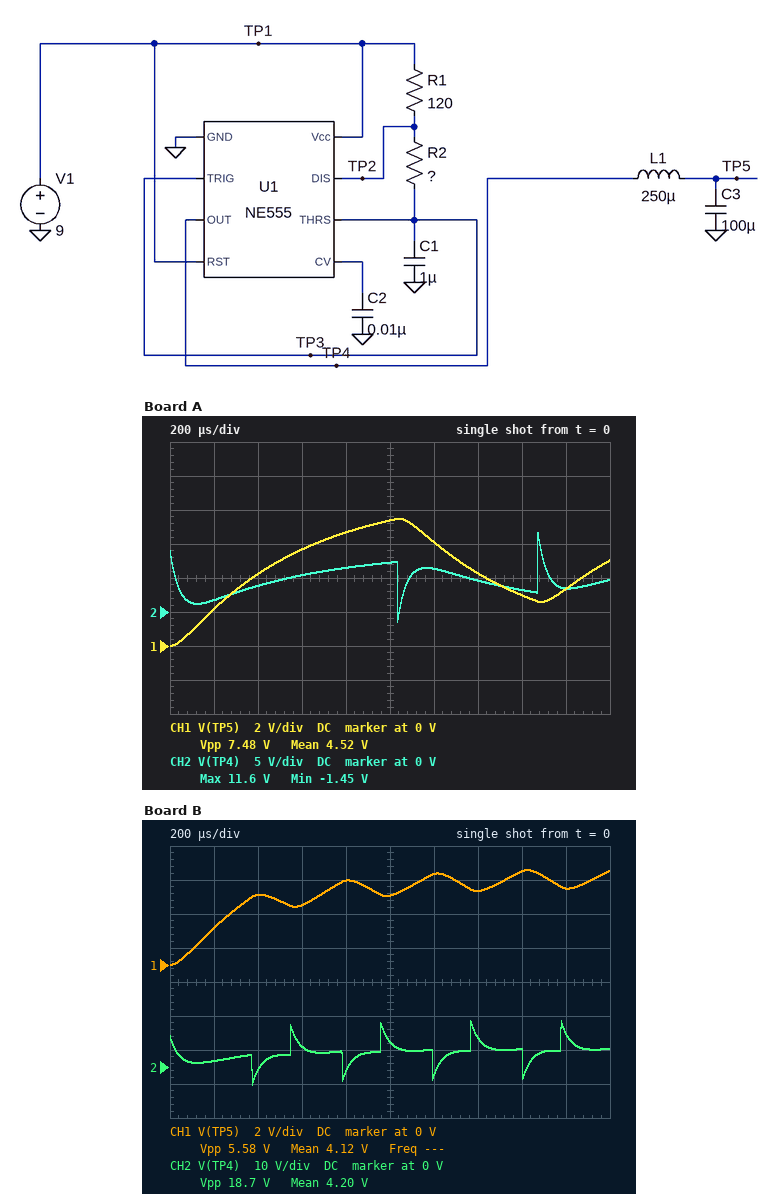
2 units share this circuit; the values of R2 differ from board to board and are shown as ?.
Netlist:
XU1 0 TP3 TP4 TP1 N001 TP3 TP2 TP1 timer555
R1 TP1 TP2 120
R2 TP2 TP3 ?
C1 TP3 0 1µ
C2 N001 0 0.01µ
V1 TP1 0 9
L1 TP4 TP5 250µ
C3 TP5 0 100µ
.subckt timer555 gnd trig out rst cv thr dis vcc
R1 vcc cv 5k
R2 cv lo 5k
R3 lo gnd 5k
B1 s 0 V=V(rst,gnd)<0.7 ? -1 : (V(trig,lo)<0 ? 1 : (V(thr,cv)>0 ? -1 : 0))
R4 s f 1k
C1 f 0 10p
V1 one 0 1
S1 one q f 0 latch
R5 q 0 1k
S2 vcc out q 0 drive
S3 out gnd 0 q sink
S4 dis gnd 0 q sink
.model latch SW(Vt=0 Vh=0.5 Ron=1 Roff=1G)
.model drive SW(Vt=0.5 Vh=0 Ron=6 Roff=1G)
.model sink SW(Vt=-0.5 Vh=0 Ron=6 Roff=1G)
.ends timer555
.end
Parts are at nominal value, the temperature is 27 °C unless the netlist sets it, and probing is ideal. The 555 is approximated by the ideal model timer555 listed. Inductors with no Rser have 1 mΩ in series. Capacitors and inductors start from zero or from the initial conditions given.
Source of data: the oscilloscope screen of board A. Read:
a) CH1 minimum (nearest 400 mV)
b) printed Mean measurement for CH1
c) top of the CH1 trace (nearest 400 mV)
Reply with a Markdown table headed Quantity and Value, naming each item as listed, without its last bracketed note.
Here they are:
| Quantity | Value |
|---|---|
| CH1 minimum | 0 V |
| printed Mean measurement for CH1 | 4.52 V |
| top of the CH1 trace | 7.6 V |
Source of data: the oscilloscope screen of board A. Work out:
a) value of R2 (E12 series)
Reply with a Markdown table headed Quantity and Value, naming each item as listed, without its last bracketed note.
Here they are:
| Quantity | Value |
|---|---|
| value of R2 | 820 Ω |
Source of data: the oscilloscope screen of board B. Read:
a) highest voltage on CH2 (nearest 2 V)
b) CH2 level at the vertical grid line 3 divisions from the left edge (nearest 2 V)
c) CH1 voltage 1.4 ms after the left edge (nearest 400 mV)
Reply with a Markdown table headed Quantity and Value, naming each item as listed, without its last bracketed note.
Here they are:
| Quantity | Value |
|---|---|
| highest voltage on CH2 | 14 V |
| CH2 level at the vertical grid line 3 divisions from the left edge | 6 V |
| CH1 voltage 1.4 ms after the left edge | 4.4 V |
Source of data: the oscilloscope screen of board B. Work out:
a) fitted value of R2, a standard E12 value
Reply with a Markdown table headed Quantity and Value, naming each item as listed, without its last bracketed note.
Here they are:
| Quantity | Value |
|---|---|
| fitted value of R2, a standard E12 value | 220 Ω |
